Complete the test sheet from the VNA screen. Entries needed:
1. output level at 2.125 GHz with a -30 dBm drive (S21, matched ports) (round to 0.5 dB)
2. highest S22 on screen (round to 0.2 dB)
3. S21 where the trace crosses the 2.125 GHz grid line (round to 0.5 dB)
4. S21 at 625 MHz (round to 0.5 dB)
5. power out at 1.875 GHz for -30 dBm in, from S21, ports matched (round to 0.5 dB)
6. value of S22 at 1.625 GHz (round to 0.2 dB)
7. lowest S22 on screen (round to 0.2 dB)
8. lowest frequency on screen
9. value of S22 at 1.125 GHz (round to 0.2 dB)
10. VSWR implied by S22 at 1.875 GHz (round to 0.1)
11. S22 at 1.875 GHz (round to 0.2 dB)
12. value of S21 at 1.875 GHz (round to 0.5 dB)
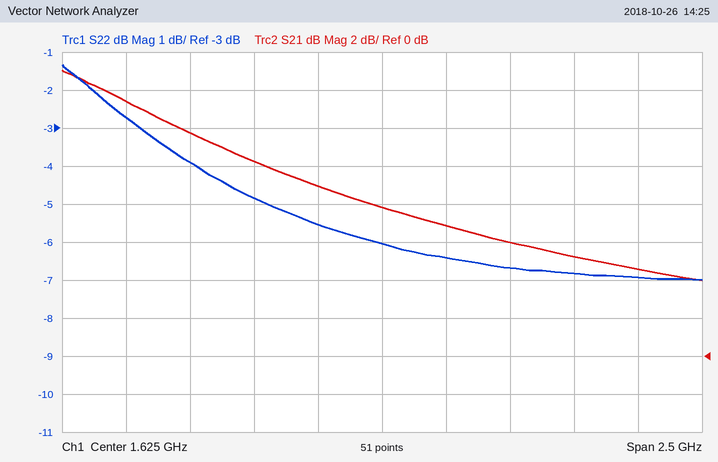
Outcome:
-24.0 dBm
-1.4 dB
6.0 dB
13.5 dB
-23.0 dBm
-6.0 dB
-7.0 dB
375 MHz
-4.8 dB
2.8
-6.4 dB
7.0 dB
